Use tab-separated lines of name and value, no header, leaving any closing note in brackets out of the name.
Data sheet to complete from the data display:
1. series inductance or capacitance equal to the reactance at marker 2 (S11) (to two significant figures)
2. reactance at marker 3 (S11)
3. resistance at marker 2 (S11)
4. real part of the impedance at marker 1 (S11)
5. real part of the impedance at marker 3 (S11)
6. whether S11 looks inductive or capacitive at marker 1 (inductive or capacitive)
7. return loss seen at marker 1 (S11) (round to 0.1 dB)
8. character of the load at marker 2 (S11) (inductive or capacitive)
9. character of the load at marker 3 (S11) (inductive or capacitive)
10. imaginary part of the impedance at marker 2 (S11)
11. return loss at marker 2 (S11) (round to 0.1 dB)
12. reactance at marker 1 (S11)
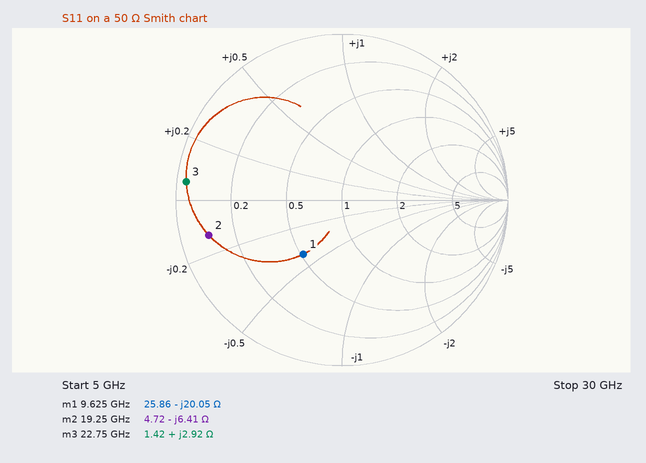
series inductance or capacitance equal to the reactance at marker 2 (S11)	1.3 pF
reactance at marker 3	+2.92 Ω
resistance at marker 2	4.72 Ω
real part of the impedance at marker 1	25.86 Ω
real part of the impedance at marker 3	1.42 Ω
whether S11 looks inductive or capacitive at marker 1	capacitive
return loss seen at marker 1 (S11)	8.0 dB
character of the load at marker 2 (S11)	capacitive
character of the load at marker 3 (S11)	inductive
imaginary part of the impedance at marker 2	-6.41 Ω
return loss at marker 2 (S11)	1.6 dB
reactance at marker 1	-20.05 Ω
